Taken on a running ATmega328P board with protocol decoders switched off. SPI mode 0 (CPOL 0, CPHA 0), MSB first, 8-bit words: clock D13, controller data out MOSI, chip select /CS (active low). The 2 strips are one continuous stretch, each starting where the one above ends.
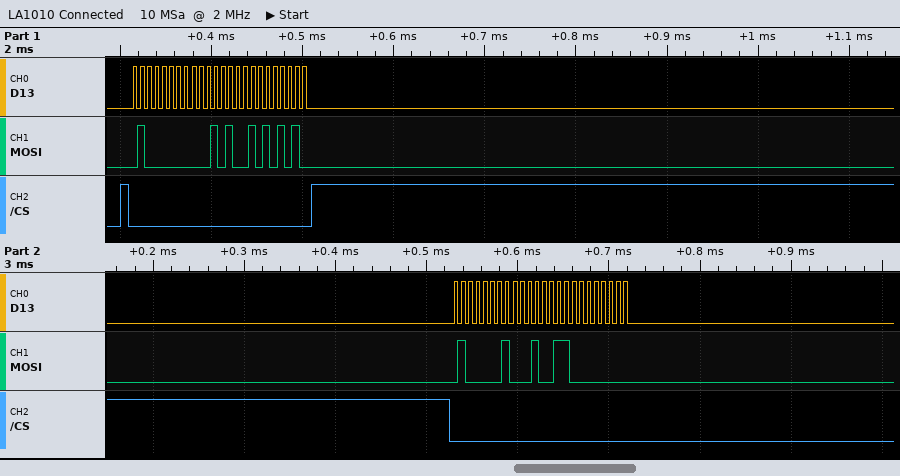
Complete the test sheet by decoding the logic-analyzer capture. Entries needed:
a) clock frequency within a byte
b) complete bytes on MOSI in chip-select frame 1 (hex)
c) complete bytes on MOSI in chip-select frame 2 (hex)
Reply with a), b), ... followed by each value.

a) 125 kHz
b) 40 14 AA
c) 41 13 00
